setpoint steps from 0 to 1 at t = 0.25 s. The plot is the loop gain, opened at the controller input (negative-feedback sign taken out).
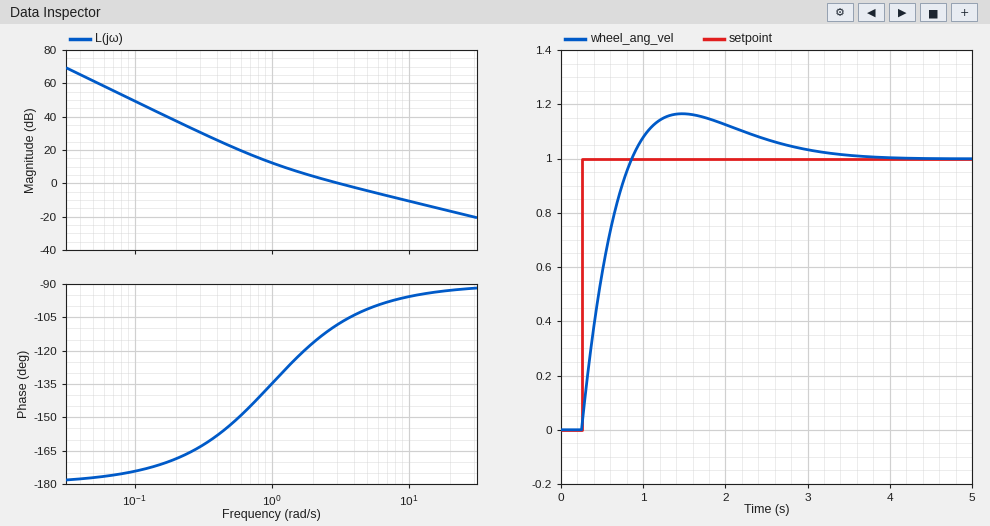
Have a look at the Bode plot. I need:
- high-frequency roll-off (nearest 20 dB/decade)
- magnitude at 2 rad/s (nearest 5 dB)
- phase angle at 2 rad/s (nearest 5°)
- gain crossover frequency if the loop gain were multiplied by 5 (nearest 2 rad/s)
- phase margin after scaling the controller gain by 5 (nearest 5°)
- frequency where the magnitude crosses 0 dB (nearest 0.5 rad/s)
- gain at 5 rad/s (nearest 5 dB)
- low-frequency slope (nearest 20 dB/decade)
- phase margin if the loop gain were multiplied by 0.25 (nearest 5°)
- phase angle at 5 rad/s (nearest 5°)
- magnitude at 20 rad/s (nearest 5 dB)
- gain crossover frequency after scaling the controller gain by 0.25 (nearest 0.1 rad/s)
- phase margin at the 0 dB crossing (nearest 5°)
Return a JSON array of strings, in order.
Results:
["-20 dB/decade", "5 dB", "-115°", "14 rad/s", "85°", "3.0 rad/s", "-5 dB", "-40 dB/decade", "45°", "-100°", "-15 dB", "1.0 rad/s", "70°"]
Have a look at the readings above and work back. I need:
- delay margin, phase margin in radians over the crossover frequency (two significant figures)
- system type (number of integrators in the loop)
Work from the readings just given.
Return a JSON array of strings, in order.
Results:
["0.41 s", "2"]
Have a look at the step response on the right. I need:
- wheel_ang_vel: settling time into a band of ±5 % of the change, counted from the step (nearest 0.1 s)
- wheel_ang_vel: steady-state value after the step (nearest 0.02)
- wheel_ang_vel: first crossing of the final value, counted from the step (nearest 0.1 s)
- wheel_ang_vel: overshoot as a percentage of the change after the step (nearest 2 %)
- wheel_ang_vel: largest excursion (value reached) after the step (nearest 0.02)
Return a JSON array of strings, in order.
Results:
["2.5 s", "1.00", "0.6 s", "16 %", "1.16"]
